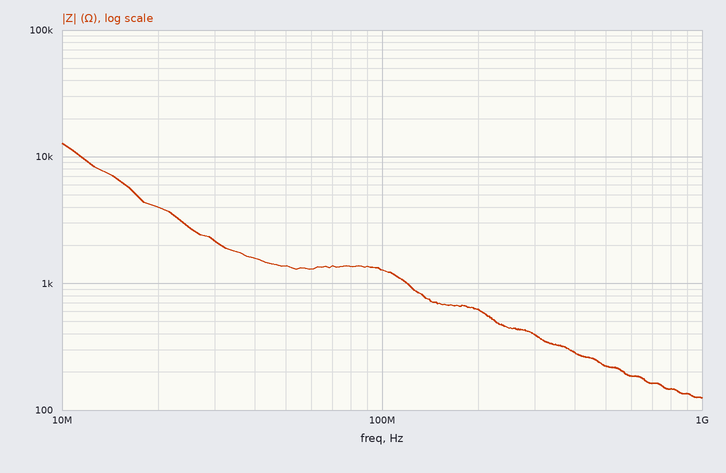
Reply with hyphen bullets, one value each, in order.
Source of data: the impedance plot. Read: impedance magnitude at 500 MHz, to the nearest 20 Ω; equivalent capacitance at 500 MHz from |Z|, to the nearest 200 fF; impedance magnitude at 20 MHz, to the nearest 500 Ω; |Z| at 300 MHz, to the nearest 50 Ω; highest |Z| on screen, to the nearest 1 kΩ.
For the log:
- 220 Ω
- 1.4 pF
- 4.0 kΩ
- 400 Ω
- 13 kΩ
